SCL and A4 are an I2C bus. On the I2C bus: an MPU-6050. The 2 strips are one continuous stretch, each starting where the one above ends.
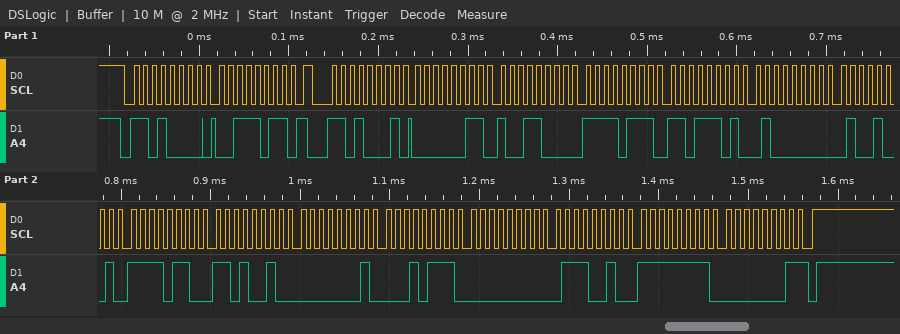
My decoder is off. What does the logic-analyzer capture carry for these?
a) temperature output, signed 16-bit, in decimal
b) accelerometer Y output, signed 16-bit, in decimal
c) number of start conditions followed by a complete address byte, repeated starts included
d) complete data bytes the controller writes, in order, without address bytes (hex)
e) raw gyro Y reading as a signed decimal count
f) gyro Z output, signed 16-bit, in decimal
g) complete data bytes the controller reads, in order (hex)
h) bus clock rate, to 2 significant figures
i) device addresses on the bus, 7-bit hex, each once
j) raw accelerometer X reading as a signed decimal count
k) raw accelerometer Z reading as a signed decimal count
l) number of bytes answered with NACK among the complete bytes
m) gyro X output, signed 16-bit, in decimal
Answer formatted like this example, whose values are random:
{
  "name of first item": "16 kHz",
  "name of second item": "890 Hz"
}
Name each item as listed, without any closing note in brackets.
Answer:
{
  "temperature output, signed 16-bit, in decimal": "-2350",
  "accelerometer Y output, signed 16-bit, in decimal": "-2083",
  "number of start conditions followed by a complete address byte, repeated starts included": "2",
  "complete data bytes the controller writes, in order, without address bytes": "3B",
  "raw gyro Y reading as a signed decimal count": "114",
  "gyro Z output, signed 16-bit, in decimal": "-255",
  "complete data bytes the controller reads, in order": "03 98 F7 DD 40 49 F6 D2 01 17 00 72 FF 01",
  "bus clock rate, to 2 significant figures": "100 kHz",
  "device addresses on the bus, 7-bit hex, each once": "0x68",
  "raw accelerometer X reading as a signed decimal count": "920",
  "raw accelerometer Z reading as a signed decimal count": "16457",
  "number of bytes answered with NACK among the complete bytes": "1",
  "gyro X output, signed 16-bit, in decimal": "279"
}
